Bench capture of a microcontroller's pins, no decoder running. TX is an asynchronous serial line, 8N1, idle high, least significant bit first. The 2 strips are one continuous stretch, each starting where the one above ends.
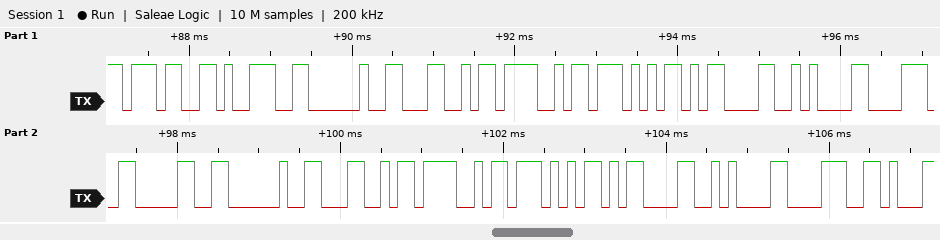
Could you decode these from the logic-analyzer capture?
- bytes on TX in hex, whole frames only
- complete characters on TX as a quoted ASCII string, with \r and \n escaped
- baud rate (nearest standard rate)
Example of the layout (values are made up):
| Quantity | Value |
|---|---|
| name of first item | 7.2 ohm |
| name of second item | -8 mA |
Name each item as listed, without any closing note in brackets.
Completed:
| Quantity | Value |
|---|---|
| bytes on TX in hex, whole frames only | 37 39 20 4C 4F 57 0D 0A 38 30 20 4C 4F 57 0D 0A 38 |
| complete characters on TX as a quoted ASCII string, with \r and \n escaped | "79 LOW\r\n80 LOW\r\n8" |
| baud rate | 9600 baud |
